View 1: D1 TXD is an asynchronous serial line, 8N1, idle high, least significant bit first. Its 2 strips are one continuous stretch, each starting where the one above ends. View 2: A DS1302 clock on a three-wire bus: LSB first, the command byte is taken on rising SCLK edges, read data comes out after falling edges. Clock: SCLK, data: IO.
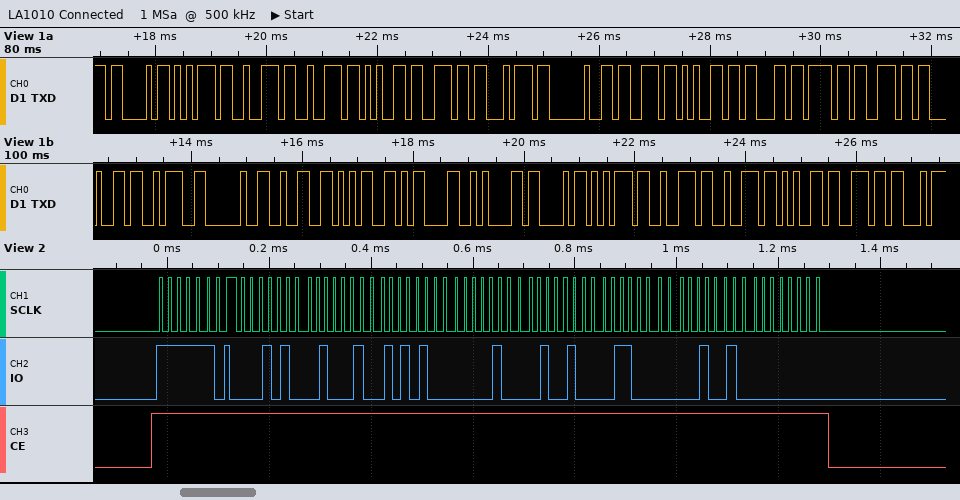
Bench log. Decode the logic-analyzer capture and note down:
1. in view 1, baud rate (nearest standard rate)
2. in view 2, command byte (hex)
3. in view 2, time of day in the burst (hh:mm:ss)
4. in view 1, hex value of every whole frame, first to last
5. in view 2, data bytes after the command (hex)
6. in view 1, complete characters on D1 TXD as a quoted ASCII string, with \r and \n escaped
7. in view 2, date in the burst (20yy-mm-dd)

9600 baud
0xBF
15:22:28
43 75 72 72 65 6E 74 20 73 65 63 6F 6E 64 3A 20 32 35 0D 0A 43 75 72 72 65 6E
28 22 15 10 12 06 24 00
"Current second: 25\r\nCurren"
2024-12-10
